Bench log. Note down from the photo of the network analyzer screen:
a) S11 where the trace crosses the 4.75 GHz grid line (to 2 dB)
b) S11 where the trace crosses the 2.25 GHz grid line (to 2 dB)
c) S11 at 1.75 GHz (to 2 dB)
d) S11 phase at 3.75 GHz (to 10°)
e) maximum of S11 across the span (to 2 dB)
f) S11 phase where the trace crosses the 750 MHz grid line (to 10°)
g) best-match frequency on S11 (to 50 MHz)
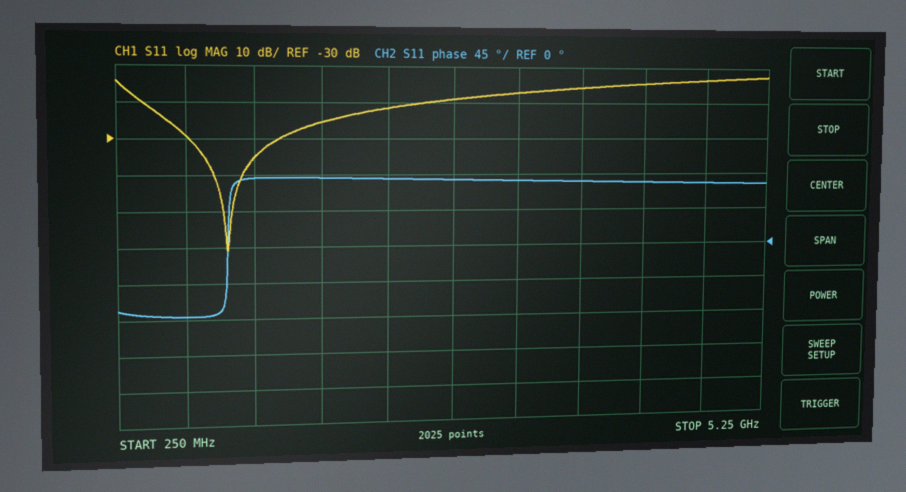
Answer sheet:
-14 dB
-22 dB
-26 dB
80°
-12 dB
-90°
1.05 GHz
